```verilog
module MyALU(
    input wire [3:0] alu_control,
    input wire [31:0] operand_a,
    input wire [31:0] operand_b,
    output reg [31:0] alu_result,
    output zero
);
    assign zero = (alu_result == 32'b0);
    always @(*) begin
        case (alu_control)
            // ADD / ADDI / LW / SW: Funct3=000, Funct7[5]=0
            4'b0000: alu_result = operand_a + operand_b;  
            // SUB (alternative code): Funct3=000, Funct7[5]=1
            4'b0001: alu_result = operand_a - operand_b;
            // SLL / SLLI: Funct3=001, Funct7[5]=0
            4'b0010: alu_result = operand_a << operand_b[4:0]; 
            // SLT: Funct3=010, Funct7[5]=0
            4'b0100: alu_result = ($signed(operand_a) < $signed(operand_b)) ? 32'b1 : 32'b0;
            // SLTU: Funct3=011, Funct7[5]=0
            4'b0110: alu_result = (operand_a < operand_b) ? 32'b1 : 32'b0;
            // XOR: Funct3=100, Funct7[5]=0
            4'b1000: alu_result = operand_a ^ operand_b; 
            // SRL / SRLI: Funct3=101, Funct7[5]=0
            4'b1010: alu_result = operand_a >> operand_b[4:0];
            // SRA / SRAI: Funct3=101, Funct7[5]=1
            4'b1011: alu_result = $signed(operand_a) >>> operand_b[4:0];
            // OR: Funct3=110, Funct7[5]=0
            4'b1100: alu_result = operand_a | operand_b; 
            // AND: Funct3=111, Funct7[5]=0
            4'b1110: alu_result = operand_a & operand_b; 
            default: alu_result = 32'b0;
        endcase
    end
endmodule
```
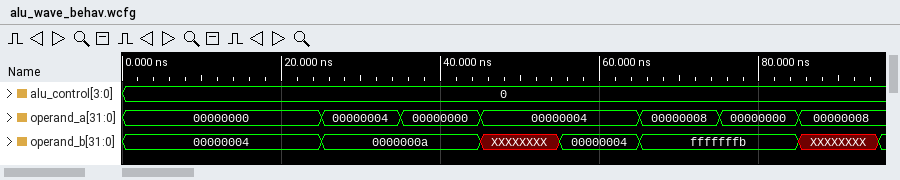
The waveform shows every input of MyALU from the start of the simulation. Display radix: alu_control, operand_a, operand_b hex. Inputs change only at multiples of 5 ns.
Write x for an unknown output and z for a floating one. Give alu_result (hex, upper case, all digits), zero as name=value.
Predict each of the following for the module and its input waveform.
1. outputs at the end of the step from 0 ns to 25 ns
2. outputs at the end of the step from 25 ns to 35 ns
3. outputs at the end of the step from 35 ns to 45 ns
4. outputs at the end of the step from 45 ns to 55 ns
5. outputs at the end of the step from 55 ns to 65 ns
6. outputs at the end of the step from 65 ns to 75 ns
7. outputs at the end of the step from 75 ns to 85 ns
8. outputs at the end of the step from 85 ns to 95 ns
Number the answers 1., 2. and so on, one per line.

1. alu_result=00000004, zero=0
2. alu_result=0000000E, zero=0
3. alu_result=0000000A, zero=0
4. alu_result=x, zero=x
5. alu_result=00000008, zero=0
6. alu_result=00000003, zero=0
7. alu_result=FFFFFFFB, zero=0
8. alu_result=x, zero=x
